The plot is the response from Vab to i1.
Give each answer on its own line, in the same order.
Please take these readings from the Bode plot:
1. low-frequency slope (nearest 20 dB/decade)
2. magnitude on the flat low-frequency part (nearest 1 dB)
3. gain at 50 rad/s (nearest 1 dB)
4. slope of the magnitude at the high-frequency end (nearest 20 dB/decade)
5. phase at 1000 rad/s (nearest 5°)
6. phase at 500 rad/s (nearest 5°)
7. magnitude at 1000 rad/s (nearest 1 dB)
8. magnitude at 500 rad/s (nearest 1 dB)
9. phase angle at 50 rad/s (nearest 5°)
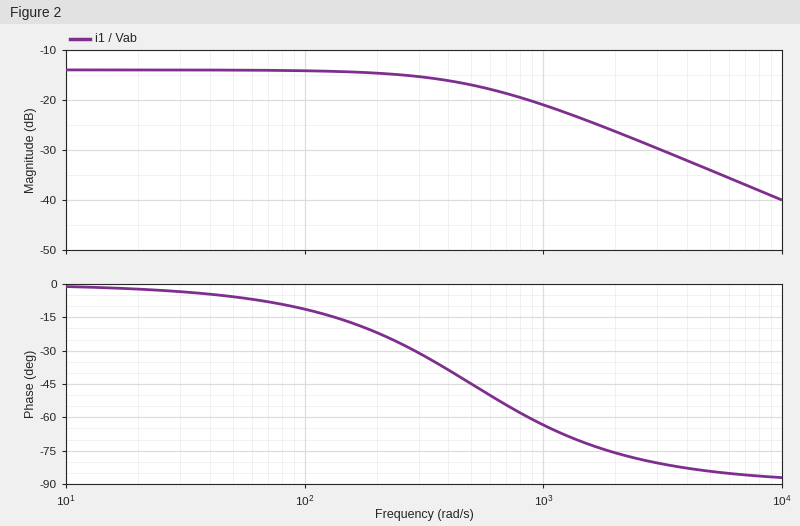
0 dB/decade
-14 dB
-14 dB
-20 dB/decade
-65°
-45°
-21 dB
-17 dB
-5°
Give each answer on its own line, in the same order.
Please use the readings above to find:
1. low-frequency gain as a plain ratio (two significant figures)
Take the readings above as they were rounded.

0.20
